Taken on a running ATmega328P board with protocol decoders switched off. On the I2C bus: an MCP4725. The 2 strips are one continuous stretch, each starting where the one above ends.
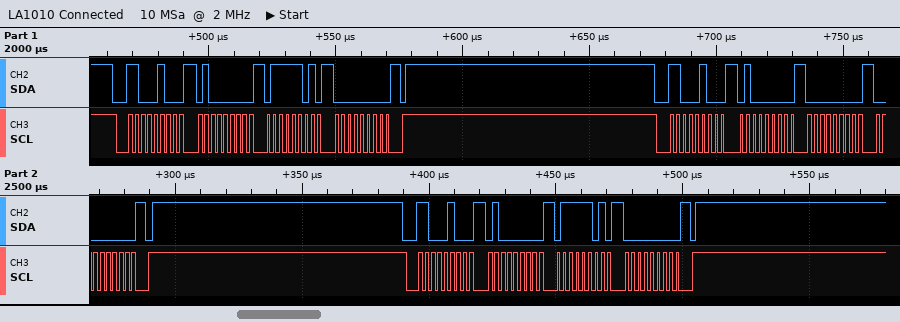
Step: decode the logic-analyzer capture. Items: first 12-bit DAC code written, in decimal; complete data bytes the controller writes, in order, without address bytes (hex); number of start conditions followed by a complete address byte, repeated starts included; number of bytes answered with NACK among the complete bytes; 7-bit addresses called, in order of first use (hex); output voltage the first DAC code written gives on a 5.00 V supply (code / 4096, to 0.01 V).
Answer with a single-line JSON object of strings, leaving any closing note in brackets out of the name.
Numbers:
{"first 12-bit DAC code written, in decimal": "2000", "complete data bytes the controller writes, in order, without address bytes": "40 7D 00 40 00 00 40 7D 00", "number of start conditions followed by a complete address byte, repeated starts included": "3", "number of bytes answered with NACK among the complete bytes": "0", "7-bit addresses called, in order of first use": "0x62", "output voltage the first DAC code written gives on a 5.00 V supply": "2.44 V"}
